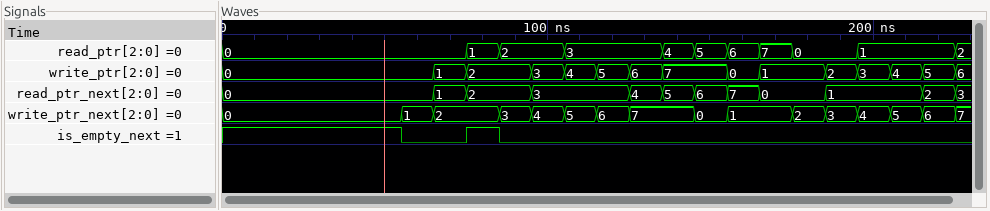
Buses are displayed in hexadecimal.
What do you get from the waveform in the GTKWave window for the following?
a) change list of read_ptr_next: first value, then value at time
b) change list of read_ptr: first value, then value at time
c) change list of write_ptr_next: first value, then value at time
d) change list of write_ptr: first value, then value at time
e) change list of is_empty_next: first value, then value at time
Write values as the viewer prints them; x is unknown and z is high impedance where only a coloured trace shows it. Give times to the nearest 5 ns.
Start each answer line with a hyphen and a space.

- 0, 1 at 65 ns, 2 at 75 ns, 3 at 95 ns, 4 at 125 ns, 5 at 135 ns, 6 at 145 ns, 7 at 155 ns, 0 at 165 ns, 1 at 185 ns, 2 at 215 ns, 3 at 225 ns
- 0, 1 at 75 ns, 2 at 85 ns, 3 at 105 ns, 4 at 135 ns, 5 at 145 ns, 6 at 155 ns, 7 at 165 ns, 0 at 175 ns, 1 at 195 ns, 2 at 225 ns
- 0, 1 at 55 ns, 2 at 65 ns, 3 at 85 ns, 4 at 95 ns, 5 at 105 ns, 6 at 115 ns, 7 at 125 ns, 0 at 145 ns, 1 at 155 ns, 2 at 175 ns, 3 at 185 ns, 4 at 195 ns, 5 at 205 ns, 6 at 215 ns, 7 at 225 ns
- 0, 1 at 65 ns, 2 at 75 ns, 3 at 95 ns, 4 at 105 ns, 5 at 115 ns, 6 at 125 ns, 7 at 135 ns, 0 at 155 ns, 1 at 165 ns, 2 at 185 ns, 3 at 195 ns, 4 at 205 ns, 5 at 215 ns, 6 at 225 ns
- 1, 0 at 55 ns, 1 at 75 ns, 0 at 85 ns
